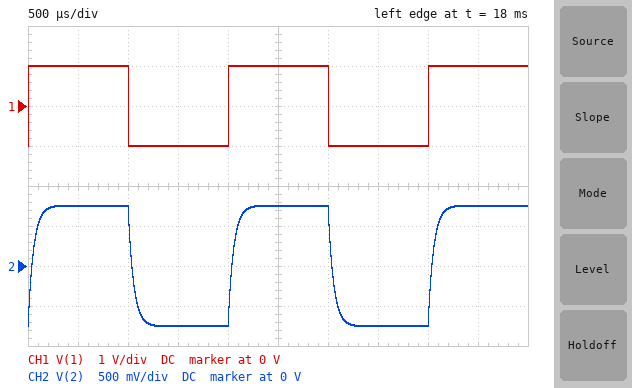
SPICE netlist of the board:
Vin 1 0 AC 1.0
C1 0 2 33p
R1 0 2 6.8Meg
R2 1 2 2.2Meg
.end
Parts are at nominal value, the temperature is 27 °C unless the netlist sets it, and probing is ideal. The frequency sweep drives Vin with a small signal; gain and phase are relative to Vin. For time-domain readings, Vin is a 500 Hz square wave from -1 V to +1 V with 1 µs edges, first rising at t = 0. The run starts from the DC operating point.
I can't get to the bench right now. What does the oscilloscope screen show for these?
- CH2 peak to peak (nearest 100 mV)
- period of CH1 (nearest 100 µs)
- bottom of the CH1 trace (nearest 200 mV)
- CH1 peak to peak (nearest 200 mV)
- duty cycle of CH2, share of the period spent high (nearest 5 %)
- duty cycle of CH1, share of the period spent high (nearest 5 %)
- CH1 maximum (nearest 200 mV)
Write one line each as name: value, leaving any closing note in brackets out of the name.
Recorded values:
CH2 peak to peak: 1.5 V
period of CH1: 2.0 ms
bottom of the CH1 trace: -1.0 V
CH1 peak to peak: 2.0 V
duty cycle of CH2, share of the period spent high: 50 %
duty cycle of CH1, share of the period spent high: 50 %
CH1 maximum: 1.0 V
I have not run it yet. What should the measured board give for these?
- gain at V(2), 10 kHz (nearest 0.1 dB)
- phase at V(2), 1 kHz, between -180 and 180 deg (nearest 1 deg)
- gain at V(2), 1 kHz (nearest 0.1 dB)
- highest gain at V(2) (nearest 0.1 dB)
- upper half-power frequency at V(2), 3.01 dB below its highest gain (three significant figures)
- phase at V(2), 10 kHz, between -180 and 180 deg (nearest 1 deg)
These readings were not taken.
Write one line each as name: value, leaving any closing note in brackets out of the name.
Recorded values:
gain at V(2), 10 kHz: -13.5 dB
phase at V(2), 1 kHz, between -180 and 180 deg: -19 deg
gain at V(2), 1 kHz: -2.9 dB
highest gain at V(2): -2.4 dB
upper half-power frequency at V(2), 3.01 dB below its highest gain: 2.90 kHz
phase at V(2), 10 kHz, between -180 and 180 deg: -74 deg
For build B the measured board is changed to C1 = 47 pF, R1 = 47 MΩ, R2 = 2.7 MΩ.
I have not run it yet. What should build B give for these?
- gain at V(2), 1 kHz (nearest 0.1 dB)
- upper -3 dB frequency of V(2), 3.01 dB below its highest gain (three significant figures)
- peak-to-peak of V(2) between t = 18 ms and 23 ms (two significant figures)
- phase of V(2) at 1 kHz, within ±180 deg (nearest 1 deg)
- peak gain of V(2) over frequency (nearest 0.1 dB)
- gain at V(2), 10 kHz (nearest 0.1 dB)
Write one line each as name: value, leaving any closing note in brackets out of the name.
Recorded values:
gain at V(2), 1 kHz: -2.4 dB
upper -3 dB frequency of V(2), 3.01 dB below its highest gain: 1.33 kHz
peak-to-peak of V(2) between t = 18 ms and 23 ms: 1.9 V
phase of V(2) at 1 kHz, within ±180 deg: -37 deg
peak gain of V(2) over frequency: -0.5 dB
gain at V(2), 10 kHz: -18.1 dB
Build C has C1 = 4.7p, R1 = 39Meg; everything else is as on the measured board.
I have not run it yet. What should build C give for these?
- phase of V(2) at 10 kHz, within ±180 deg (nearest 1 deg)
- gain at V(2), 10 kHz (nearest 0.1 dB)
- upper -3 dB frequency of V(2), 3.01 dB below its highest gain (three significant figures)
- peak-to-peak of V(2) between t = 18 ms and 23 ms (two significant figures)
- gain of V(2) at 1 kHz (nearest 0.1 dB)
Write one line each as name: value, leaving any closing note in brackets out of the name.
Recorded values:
phase of V(2) at 10 kHz, within ±180 deg: -32 deg
gain at V(2), 10 kHz: -1.9 dB
upper -3 dB frequency of V(2), 3.01 dB below its highest gain: 16.3 kHz
peak-to-peak of V(2) between t = 18 ms and 23 ms: 1.9 V
gain of V(2) at 1 kHz: -0.5 dB
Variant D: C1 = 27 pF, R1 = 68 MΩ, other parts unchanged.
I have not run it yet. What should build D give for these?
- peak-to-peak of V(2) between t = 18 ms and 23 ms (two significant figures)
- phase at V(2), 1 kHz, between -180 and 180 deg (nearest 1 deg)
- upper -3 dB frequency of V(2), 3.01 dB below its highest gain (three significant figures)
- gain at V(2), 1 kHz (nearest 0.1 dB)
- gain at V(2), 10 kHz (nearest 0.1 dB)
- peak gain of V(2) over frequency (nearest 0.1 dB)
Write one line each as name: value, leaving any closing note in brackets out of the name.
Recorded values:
peak-to-peak of V(2) between t = 18 ms and 23 ms: 1.9 V
phase at V(2), 1 kHz, between -180 and 180 deg: -20 deg
upper -3 dB frequency of V(2), 3.01 dB below its highest gain: 2.77 kHz
gain at V(2), 1 kHz: -0.8 dB
gain at V(2), 10 kHz: -11.8 dB
peak gain of V(2) over frequency: -0.3 dB
